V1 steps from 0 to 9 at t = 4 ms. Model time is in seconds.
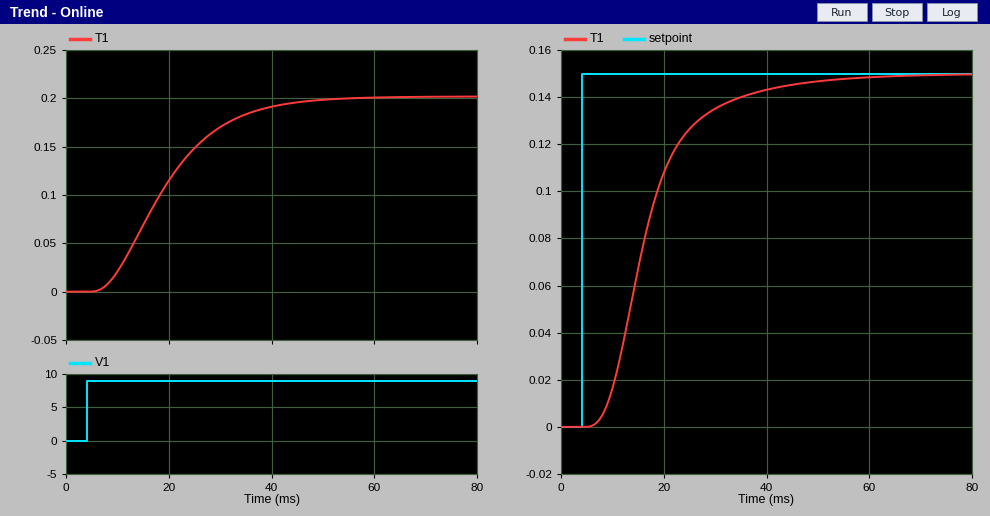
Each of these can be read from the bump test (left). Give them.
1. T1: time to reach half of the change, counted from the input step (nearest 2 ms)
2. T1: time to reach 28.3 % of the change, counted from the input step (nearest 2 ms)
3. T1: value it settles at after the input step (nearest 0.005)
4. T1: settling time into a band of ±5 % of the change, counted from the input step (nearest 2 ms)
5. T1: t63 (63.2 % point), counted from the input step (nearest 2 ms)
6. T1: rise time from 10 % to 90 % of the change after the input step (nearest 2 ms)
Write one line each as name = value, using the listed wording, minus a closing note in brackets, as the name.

T1: time to reach half of the change, counted from the input step = 14 ms
T1: time to reach 28.3 % of the change, counted from the input step = 10 ms
T1: value it settles at after the input step = 0.200
T1: settling time into a band of ±5 % of the change, counted from the input step = 36 ms
T1: t63 (63.2 % point), counted from the input step = 18 ms
T1: rise time from 10 % to 90 % of the change after the input step = 24 ms
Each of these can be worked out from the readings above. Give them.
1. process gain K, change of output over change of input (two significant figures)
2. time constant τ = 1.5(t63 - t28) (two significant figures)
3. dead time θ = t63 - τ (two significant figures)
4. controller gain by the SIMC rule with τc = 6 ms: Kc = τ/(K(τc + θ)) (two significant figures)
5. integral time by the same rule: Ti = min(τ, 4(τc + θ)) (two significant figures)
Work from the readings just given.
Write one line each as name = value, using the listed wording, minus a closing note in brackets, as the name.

process gain K, change of output over change of input = 0.022
time constant τ = 1.5(t63 - t28) = 12 ms
dead time θ = t63 - τ = 6.0 ms
controller gain by the SIMC rule with τc = 6 ms: Kc = τ/(K(τc + θ)) = 45
integral time by the same rule: Ti = min(τ, 4(τc + θ)) = 12 ms
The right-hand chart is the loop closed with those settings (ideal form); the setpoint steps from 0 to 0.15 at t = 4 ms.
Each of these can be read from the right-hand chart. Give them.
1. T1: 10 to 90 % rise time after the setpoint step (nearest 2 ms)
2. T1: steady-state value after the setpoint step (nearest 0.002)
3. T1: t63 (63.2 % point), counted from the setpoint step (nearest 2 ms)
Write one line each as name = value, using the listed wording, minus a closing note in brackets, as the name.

T1: 10 to 90 % rise time after the setpoint step = 20 ms
T1: steady-state value after the setpoint step = 0.150
T1: t63 (63.2 % point), counted from the setpoint step = 14 ms
